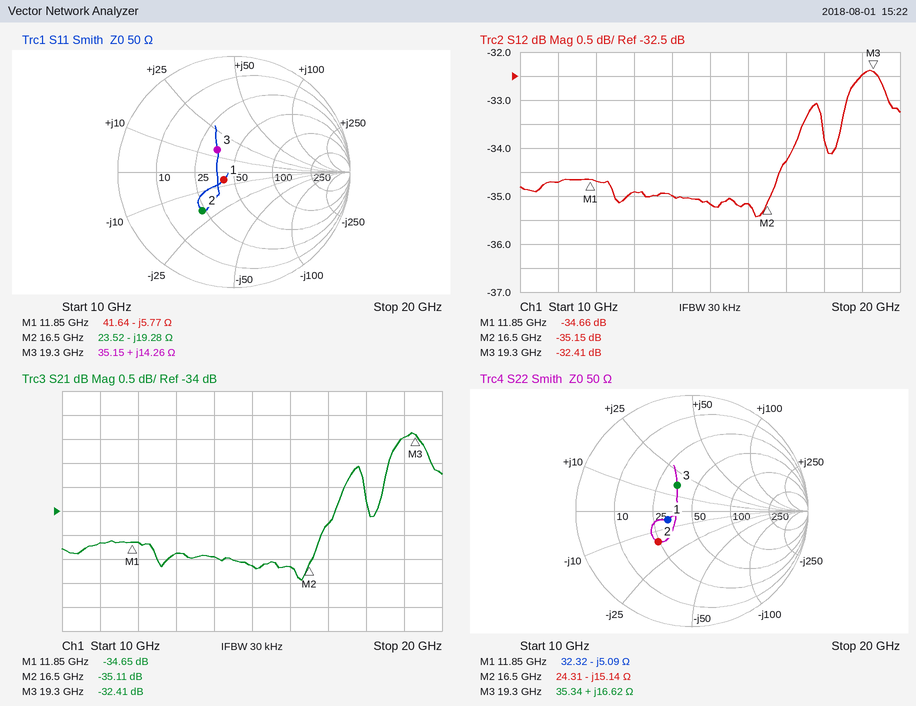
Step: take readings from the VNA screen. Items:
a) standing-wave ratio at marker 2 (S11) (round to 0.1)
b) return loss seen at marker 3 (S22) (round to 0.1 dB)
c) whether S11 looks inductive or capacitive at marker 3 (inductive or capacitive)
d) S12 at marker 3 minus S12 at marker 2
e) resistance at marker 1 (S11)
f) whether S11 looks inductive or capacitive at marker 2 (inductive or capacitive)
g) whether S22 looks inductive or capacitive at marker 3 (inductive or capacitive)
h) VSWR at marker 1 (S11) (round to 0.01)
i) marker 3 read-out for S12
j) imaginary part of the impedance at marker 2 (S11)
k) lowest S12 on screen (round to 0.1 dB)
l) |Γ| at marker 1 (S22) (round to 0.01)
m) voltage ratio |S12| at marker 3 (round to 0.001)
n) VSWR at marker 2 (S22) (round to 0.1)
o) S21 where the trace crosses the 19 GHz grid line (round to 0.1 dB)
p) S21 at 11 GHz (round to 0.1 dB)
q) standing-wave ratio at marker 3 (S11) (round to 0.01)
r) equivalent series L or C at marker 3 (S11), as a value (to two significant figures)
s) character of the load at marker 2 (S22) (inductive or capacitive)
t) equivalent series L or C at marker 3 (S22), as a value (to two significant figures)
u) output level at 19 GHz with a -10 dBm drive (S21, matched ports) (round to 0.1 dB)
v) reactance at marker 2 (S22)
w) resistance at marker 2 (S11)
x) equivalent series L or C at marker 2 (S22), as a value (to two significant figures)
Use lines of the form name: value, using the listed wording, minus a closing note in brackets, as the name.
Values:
standing-wave ratio at marker 2 (S11): 2.5
return loss seen at marker 3 (S22): 11.9 dB
whether S11 looks inductive or capacitive at marker 3: inductive
S12 at marker 3 minus S12 at marker 2: 2.74 dB
resistance at marker 1: 41.64 Ω
whether S11 looks inductive or capacitive at marker 2: capacitive
whether S22 looks inductive or capacitive at marker 3: inductive
VSWR at marker 1 (S11): 1.25
marker 3 read-out for S12: -32.41 dB
imaginary part of the impedance at marker 2: -19.28 Ω
lowest S12 on screen: -35.4 dB
|Γ| at marker 1 (S22): 0.22
voltage ratio |S12| at marker 3: 0.024
VSWR at marker 2 (S22): 2.3
S21 where the trace crosses the 19 GHz grid line: -32.5 dB
S21 at 11 GHz: -34.7 dB
standing-wave ratio at marker 3 (S11): 1.63
equivalent series L or C at marker 3 (S11), as a value: 120 pH
character of the load at marker 2 (S22): capacitive
equivalent series L or C at marker 3 (S22), as a value: 140 pH
output level at 19 GHz with a -10 dBm drive (S21, matched ports): -42.5 dBm
reactance at marker 2: -15.14 Ω
resistance at marker 2: 23.52 Ω
equivalent series L or C at marker 2 (S22), as a value: 640 fF
